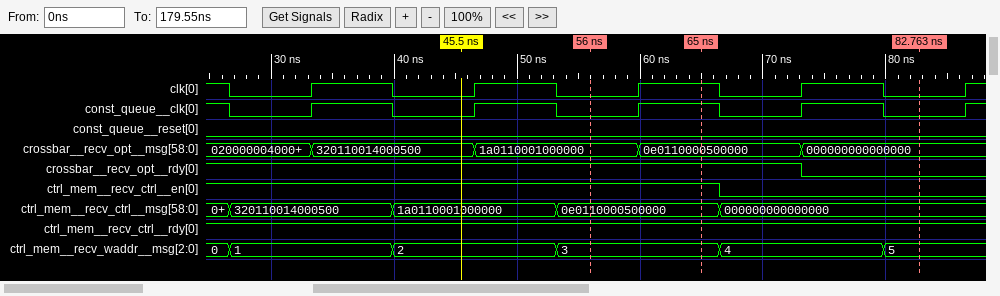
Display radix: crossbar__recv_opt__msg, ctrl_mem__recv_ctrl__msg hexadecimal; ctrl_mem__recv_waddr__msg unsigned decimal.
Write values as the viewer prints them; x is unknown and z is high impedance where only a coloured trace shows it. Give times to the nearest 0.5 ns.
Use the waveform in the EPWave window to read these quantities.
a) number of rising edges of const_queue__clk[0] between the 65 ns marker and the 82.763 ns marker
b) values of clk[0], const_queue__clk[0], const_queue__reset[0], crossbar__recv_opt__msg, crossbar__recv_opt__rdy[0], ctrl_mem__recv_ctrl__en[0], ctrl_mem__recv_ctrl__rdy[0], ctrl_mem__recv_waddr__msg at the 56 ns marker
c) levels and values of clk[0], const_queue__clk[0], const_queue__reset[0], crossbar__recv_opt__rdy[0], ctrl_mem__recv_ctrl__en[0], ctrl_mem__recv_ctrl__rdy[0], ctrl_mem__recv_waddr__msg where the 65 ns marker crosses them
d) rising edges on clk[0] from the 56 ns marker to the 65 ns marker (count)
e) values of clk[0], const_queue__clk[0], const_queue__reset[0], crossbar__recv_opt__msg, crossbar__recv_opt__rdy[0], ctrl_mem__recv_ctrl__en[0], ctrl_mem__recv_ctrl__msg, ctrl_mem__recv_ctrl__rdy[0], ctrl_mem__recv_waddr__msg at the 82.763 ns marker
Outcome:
1
clk[0]=0, const_queue__clk[0]=0, const_queue__reset[0]=0, crossbar__recv_opt__msg=1a0110001000000, crossbar__recv_opt__rdy[0]=1, ctrl_mem__recv_ctrl__en[0]=1, ctrl_mem__recv_ctrl__rdy[0]=1, ctrl_mem__recv_waddr__msg=3
clk[0]=1, const_queue__clk[0]=1, const_queue__reset[0]=0, crossbar__recv_opt__rdy[0]=1, ctrl_mem__recv_ctrl__en[0]=1, ctrl_mem__recv_ctrl__rdy[0]=1, ctrl_mem__recv_waddr__msg=3
1
clk[0]=0, const_queue__clk[0]=0, const_queue__reset[0]=0, crossbar__recv_opt__msg=000000000000000, crossbar__recv_opt__rdy[0]=0, ctrl_mem__recv_ctrl__en[0]=0, ctrl_mem__recv_ctrl__msg=000000000000000, ctrl_mem__recv_ctrl__rdy[0]=1, ctrl_mem__recv_waddr__msg=5
